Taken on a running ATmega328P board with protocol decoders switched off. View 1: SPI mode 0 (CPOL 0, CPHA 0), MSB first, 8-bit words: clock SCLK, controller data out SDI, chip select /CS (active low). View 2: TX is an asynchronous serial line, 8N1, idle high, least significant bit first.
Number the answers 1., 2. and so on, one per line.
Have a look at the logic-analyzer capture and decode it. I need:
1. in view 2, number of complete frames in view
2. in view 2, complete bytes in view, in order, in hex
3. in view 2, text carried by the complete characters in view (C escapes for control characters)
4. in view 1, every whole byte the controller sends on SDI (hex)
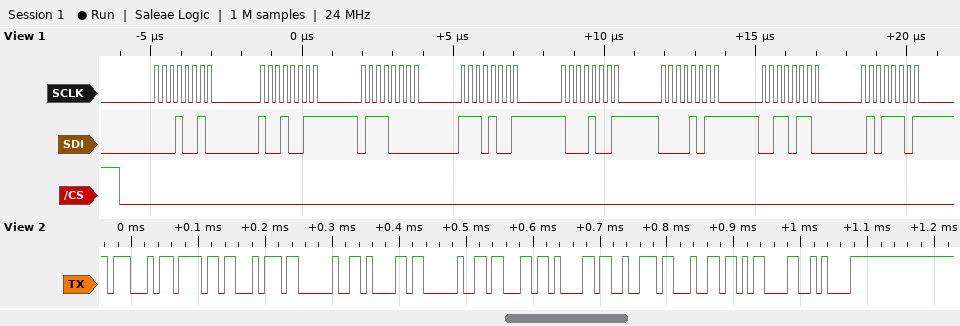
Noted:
1. 12
2. 47 6F 74 20 61 20 63 61 72 64 0D 0A
3. "Got a card\r\n"
4. 12 93 70 E9 89 0B 36 5D
